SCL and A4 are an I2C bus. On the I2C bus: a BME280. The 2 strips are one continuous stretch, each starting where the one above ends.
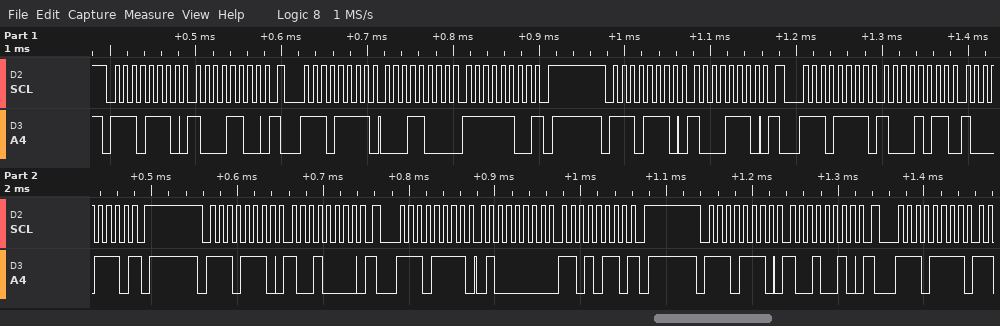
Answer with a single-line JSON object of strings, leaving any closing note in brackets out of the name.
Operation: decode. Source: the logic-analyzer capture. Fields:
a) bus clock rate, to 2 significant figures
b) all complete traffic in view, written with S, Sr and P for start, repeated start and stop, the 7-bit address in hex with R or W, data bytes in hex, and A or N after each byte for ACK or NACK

{"bus clock rate, to 2 significant figures": "100 kHz", "all complete traffic in view, written with S, Sr and P for start, repeated start and stop, the 7-bit address in hex with R or W, data bytes in hex, and A or N after each byte for ACK or NACK": "S 77W A 8C A Sr 77R A 18 A FC N P S 77W A 8E A Sr 77R A 8B A 8E N P S 77W A 90 A Sr 77R A 40 A D6 N P S 77W A 92 A Sr 77R A"}
